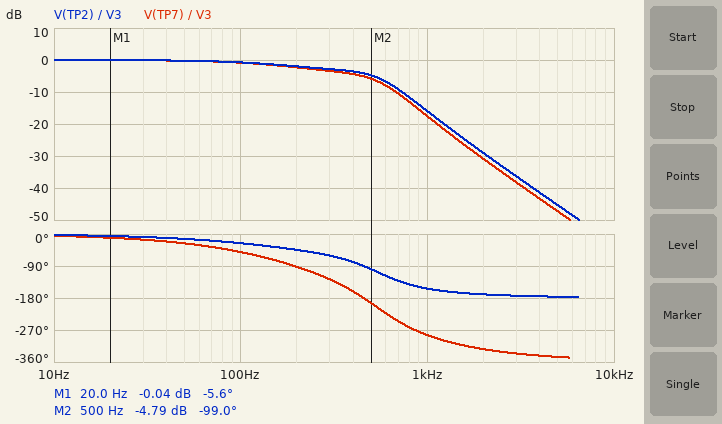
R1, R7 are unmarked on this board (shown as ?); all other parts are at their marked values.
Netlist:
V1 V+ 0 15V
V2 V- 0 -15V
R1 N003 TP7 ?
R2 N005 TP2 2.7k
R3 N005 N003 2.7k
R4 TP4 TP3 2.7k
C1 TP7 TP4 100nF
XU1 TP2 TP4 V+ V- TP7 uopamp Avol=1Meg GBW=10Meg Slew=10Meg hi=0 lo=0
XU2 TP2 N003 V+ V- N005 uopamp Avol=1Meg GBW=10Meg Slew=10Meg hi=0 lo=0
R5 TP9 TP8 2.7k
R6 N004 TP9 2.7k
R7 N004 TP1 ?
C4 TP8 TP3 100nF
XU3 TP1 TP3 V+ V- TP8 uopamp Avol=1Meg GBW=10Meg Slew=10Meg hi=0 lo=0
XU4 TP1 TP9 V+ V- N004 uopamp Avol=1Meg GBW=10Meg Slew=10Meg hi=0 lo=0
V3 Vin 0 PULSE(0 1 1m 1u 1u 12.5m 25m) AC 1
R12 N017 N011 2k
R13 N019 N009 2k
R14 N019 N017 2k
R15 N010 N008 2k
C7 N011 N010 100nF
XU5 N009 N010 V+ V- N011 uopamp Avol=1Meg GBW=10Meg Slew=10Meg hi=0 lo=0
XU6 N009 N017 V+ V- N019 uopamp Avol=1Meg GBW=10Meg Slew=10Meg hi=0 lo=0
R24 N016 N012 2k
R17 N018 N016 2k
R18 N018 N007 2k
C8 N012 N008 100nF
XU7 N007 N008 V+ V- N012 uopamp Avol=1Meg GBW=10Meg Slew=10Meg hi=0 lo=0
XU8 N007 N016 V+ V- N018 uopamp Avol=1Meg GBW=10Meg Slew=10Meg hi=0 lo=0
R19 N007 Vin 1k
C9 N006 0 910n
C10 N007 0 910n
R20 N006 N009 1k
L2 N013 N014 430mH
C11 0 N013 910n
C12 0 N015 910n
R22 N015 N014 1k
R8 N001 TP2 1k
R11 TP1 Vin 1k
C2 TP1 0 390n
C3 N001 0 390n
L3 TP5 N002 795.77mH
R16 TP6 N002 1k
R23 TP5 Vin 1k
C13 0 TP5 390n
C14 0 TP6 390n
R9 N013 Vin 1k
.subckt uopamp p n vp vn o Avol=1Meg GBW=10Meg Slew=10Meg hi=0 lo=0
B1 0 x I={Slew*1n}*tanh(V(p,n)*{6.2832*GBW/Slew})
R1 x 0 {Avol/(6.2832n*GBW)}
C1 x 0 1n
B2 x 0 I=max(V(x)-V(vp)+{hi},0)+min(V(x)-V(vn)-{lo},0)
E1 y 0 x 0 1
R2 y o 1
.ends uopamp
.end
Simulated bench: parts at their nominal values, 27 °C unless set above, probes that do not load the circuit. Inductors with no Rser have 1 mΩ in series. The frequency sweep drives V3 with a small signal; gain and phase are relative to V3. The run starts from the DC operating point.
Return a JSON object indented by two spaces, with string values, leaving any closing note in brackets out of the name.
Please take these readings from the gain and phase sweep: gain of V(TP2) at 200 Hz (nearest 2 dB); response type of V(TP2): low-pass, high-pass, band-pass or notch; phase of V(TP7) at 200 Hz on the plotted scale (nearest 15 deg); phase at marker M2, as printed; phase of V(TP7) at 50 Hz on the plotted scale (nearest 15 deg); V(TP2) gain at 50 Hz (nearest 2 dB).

{
  "gain of V(TP2) at 200 Hz": "-2 dB",
  "response type of V(TP2): low-pass, high-pass, band-pass or notch": "low-pass",
  "phase of V(TP7) at 200 Hz on the plotted scale": "-90 deg",
  "phase at marker M2, as printed": "-99.0 deg",
  "phase of V(TP7) at 50 Hz on the plotted scale": "-30 deg",
  "V(TP2) gain at 50 Hz": "0 dB"
}
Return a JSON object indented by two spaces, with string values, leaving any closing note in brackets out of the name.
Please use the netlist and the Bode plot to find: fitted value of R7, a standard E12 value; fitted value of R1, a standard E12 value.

{
  "fitted value of R7, a standard E12 value": "1.8 kΩ",
  "fitted value of R1, a standard E12 value": "1.8 kΩ"
}
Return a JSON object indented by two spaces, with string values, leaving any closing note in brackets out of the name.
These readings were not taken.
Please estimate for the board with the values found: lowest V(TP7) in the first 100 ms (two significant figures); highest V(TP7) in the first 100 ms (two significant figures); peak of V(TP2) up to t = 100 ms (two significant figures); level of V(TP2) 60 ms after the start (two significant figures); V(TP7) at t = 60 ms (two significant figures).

{
  "lowest V(TP7) in the first 100 ms": "-77 mV",
  "highest V(TP7) in the first 100 ms": "1.1 V",
  "peak of V(TP2) up to t = 100 ms": "1.0 V",
  "level of V(TP2) 60 ms after the start": "1.0 V",
  "V(TP7) at t = 60 ms": "1.0 V"
}
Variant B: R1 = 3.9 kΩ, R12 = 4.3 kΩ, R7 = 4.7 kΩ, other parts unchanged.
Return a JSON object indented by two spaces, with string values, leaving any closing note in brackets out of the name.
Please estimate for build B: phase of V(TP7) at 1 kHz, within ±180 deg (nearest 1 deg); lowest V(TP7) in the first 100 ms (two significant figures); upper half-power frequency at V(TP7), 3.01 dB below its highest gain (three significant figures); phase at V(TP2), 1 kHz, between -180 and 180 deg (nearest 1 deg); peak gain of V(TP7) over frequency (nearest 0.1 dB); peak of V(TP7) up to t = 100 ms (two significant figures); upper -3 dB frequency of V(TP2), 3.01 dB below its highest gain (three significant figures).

{
  "phase of V(TP7) at 1 kHz, within ±180 deg": "41 deg",
  "lowest V(TP7) in the first 100 ms": "-510 mV",
  "upper half-power frequency at V(TP7), 3.01 dB below its highest gain": "390 Hz",
  "phase at V(TP2), 1 kHz, between -180 and 180 deg": "-169 deg",
  "peak gain of V(TP7) over frequency": "4.8 dB",
  "peak of V(TP7) up to t = 100 ms": "1.5 V",
  "upper -3 dB frequency of V(TP2), 3.01 dB below its highest gain": "342 Hz"
}
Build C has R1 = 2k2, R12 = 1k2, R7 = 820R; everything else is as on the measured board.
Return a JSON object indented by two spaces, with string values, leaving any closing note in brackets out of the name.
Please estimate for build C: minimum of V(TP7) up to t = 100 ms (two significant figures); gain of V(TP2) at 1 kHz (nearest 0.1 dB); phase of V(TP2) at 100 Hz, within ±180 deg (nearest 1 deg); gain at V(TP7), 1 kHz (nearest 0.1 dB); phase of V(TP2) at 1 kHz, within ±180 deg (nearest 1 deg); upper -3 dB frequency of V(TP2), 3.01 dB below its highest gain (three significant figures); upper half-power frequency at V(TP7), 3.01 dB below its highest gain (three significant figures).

{
  "minimum of V(TP7) up to t = 100 ms": "-130 mV",
  "gain of V(TP2) at 1 kHz": "-16.6 dB",
  "phase of V(TP2) at 100 Hz, within ±180 deg": "-39 deg",
  "gain at V(TP7), 1 kHz": "-15.2 dB",
  "phase of V(TP2) at 1 kHz, within ±180 deg": "-150 deg",
  "upper -3 dB frequency of V(TP2), 3.01 dB below its highest gain": "108 Hz",
  "upper half-power frequency at V(TP7), 3.01 dB below its highest gain": "111 Hz"
}
